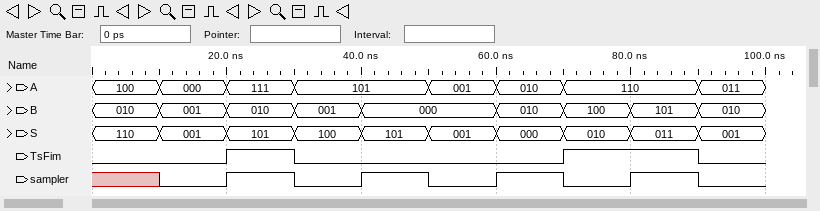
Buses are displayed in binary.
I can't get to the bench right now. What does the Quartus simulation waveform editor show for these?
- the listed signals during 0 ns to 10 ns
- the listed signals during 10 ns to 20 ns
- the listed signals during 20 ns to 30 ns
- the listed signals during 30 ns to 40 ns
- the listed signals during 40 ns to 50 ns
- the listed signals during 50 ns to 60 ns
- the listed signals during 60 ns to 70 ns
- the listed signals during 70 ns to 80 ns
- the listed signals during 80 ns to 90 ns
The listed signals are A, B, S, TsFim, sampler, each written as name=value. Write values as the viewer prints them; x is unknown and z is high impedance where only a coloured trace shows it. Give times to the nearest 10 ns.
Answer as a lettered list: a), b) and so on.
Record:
a) A=100, B=010, S=110, TsFim=0, sampler=x
b) A=000, B=001, S=001, TsFim=0, sampler=0
c) A=111, B=010, S=101, TsFim=1, sampler=1
d) A=101, B=001, S=100, TsFim=0, sampler=0
e) A=101, B=000, S=101, TsFim=0, sampler=1
f) A=001, B=000, S=001, TsFim=0, sampler=0
g) A=010, B=010, S=000, TsFim=0, sampler=1
h) A=110, B=100, S=010, TsFim=1, sampler=0
i) A=110, B=101, S=011, TsFim=1, sampler=1
